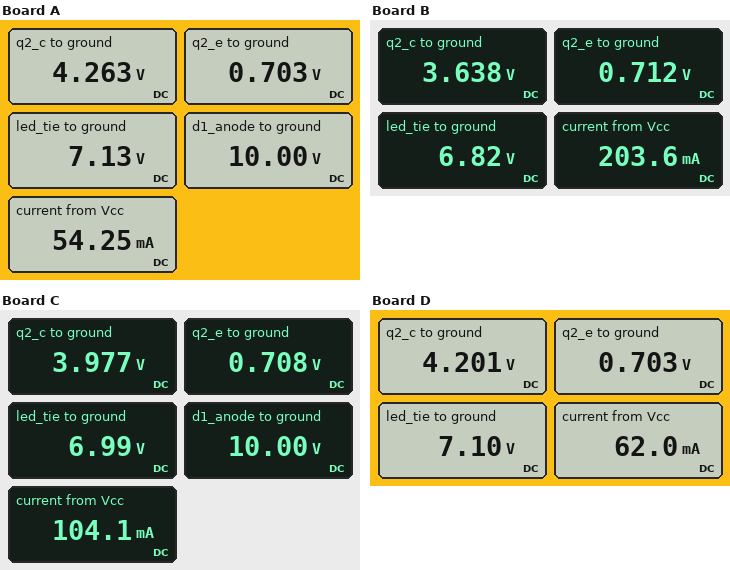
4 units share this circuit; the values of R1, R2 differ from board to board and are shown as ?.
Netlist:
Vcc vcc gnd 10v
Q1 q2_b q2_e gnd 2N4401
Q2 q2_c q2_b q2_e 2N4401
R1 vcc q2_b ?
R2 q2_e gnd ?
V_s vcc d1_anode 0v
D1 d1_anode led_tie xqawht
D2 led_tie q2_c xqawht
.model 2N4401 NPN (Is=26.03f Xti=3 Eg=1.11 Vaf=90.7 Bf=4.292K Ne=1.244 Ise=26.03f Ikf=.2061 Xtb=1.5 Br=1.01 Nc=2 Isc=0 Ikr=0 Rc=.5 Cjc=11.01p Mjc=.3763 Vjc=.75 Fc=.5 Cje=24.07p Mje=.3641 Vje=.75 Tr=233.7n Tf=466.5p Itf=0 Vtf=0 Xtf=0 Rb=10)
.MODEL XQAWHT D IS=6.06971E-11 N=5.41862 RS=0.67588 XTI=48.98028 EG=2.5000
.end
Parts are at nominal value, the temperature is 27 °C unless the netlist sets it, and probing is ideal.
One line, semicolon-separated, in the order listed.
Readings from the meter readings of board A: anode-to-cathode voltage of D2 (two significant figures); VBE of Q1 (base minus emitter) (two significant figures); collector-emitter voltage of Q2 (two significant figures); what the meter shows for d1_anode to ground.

2.9 V; 700 mV; 3.6 V; 10.00 V
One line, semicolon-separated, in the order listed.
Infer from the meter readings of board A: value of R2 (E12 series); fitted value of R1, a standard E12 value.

18 Ω; 560 Ω
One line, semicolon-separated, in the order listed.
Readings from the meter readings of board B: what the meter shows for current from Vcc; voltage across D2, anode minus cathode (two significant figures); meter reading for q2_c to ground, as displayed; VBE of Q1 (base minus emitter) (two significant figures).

203.6 mA; 3.2 V; 3.638 V; 710 mV
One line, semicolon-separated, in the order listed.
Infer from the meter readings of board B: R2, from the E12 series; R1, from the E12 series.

3.9 Ω; 390 Ω
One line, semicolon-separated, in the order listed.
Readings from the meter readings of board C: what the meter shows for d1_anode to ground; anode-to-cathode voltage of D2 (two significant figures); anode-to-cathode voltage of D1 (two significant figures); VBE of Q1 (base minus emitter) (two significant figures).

10.00 V; 3.0 V; 3.0 V; 710 mV
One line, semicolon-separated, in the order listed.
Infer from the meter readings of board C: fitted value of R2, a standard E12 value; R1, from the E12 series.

8.2 Ω; 470 Ω
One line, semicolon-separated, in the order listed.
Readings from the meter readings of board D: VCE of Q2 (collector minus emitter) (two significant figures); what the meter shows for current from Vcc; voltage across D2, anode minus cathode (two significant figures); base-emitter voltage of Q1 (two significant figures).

3.5 V; 62.0 mA; 2.9 V; 700 mV
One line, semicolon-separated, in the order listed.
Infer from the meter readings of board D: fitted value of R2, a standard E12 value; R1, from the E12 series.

15 Ω; 560 Ω
